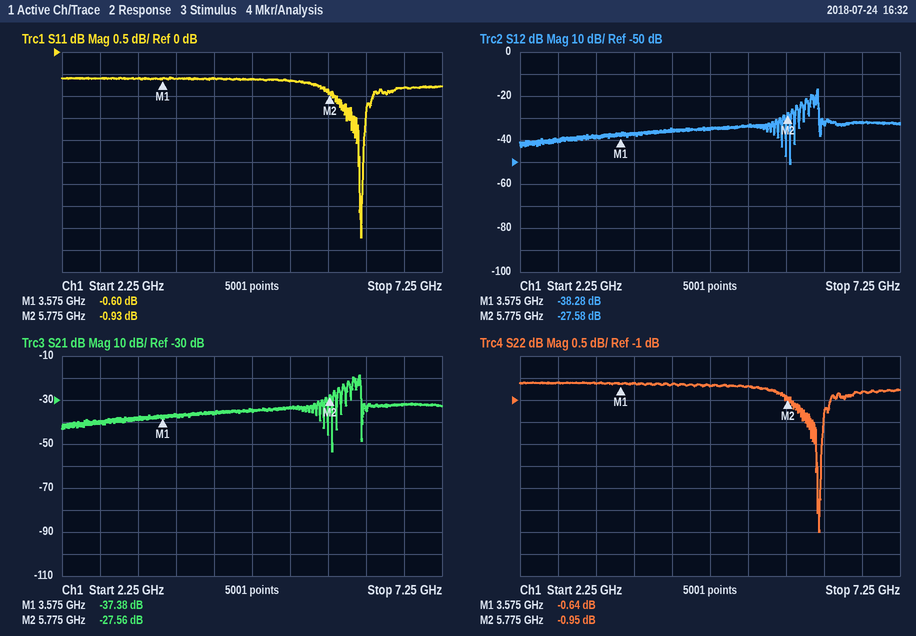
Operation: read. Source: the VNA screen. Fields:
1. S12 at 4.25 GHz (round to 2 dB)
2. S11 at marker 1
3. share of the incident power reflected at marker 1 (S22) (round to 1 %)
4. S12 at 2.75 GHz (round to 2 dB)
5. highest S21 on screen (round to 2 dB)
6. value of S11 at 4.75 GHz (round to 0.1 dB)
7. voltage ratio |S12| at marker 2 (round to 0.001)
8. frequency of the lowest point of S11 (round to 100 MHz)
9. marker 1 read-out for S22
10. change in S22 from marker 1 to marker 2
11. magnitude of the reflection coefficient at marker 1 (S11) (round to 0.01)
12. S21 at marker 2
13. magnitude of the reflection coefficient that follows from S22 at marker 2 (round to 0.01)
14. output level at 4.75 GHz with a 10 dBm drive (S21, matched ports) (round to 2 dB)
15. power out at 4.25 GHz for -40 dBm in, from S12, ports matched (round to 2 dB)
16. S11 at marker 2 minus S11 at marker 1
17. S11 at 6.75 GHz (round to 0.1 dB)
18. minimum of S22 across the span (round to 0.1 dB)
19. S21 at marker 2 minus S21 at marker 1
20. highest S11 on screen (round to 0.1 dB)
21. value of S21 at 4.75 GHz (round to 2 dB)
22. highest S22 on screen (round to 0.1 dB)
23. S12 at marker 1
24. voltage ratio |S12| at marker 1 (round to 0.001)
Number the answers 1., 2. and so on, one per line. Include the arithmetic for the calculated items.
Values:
1. -36 dB
2. -0.60 dB
3. 10^(-0.64/10) ≈ 86 %
4. -40 dB
5. -18 dB
6. -0.6 dB
7. 10^(-27.58/20) ≈ 0.042
8. 6.2 GHz
9. -0.64 dB
10. -0.95 − (-0.64) = -0.31 dB
11. 10^(-0.6/20) ≈ 0.93
12. -27.56 dB
13. 10^(-0.95/20) ≈ 0.90
14. 10 dBm + (-34 dB) = -24 dBm
15. -40 dBm + (-36 dB) = -76 dBm
16. -0.93 − (-0.6) = -0.33 dB
17. -0.8 dB
18. -4.0 dB
19. -27.56 − (-37.38) = 9.82 dB
20. -0.6 dB
21. -34 dB
22. -0.6 dB
23. -38.28 dB
24. 10^(-38.28/20) ≈ 0.012
